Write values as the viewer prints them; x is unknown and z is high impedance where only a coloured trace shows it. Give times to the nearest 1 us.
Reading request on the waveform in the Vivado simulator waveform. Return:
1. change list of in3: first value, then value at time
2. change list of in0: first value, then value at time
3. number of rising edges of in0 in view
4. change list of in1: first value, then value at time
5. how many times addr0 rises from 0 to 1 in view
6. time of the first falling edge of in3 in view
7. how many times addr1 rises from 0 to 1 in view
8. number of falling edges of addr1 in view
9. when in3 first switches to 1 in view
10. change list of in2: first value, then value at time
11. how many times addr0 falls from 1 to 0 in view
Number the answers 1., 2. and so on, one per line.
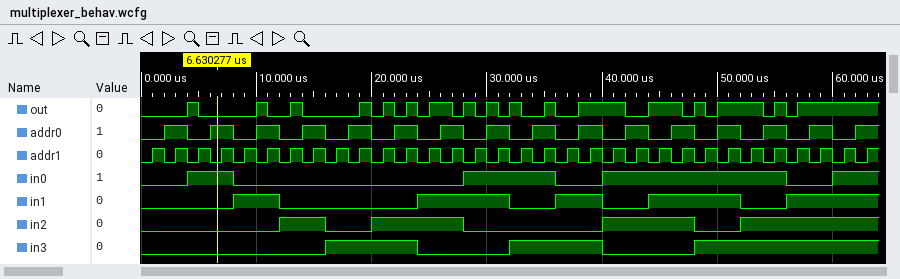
1. 0, 1 at 16 us, 0 at 24 us, 1 at 32 us, 0 at 40 us, 1 at 48 us
2. 0, 1 at 4 us, 0 at 8 us, 1 at 28 us, 0 at 36 us, 1 at 40 us, 0 at 56 us, 1 at 60 us
3. 4
4. 0, 1 at 8 us, 0 at 12 us, 1 at 24 us, 0 at 32 us, 1 at 36 us, 0 at 40 us, 1 at 44 us, 0 at 52 us, 1 at 56 us
5. 16
6. 24 us
7. 32
8. 31
9. 16 us
10. 0, 1 at 12 us, 0 at 16 us, 1 at 20 us, 0 at 28 us, 1 at 40 us, 0 at 48 us, 1 at 52 us
11. 15
